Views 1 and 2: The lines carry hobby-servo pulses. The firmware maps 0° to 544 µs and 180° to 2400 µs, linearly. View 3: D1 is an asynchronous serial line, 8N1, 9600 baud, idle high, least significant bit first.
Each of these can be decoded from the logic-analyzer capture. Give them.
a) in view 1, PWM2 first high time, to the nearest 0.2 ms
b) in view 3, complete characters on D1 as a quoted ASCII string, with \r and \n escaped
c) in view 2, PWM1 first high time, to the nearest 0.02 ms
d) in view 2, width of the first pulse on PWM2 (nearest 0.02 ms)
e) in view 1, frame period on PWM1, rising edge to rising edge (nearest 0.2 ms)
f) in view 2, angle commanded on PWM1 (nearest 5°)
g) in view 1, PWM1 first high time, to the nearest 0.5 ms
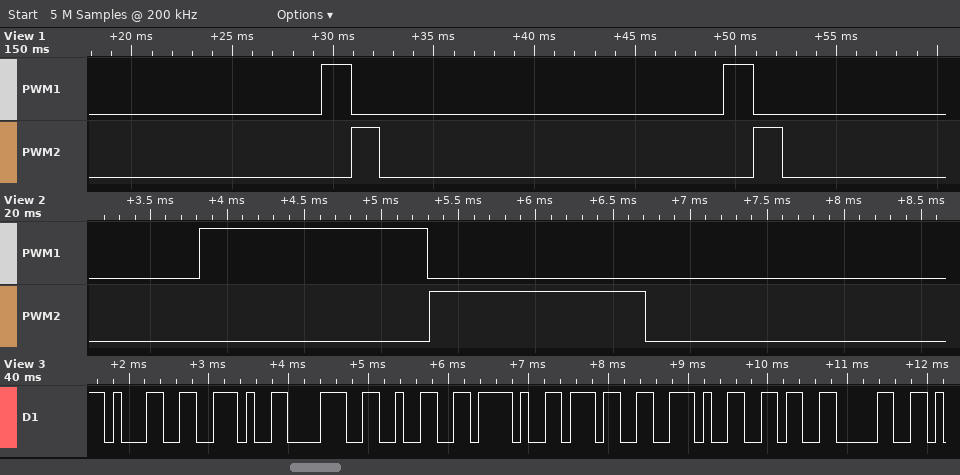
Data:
1.4 ms
"1.82/7.60"
1.48 ms
1.40 ms
20.0 ms
90°
1.5 ms
